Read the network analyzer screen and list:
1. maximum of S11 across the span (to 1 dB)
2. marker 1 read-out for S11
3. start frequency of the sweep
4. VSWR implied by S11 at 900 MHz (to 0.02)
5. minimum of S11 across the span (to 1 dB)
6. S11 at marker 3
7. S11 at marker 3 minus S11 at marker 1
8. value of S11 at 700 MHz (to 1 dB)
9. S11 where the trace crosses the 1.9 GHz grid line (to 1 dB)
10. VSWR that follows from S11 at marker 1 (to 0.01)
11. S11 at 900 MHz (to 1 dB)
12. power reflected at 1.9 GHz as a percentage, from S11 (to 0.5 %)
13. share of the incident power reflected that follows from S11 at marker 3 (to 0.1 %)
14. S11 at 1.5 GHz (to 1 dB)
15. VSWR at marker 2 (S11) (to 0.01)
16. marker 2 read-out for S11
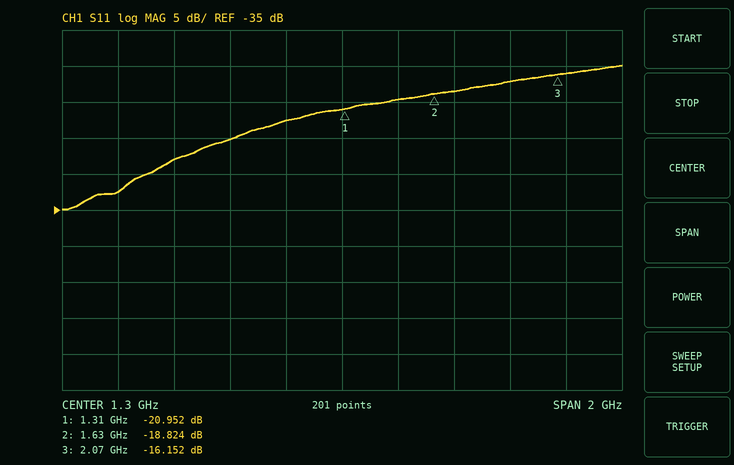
-15 dB
-20.952 dB
300 MHz
1.12
-35 dB
-16.152 dB
4.800 dB
-28 dB
-17 dB
1.20
-25 dB
2.0 %
2.4 %
-20 dB
1.26
-18.824 dB
